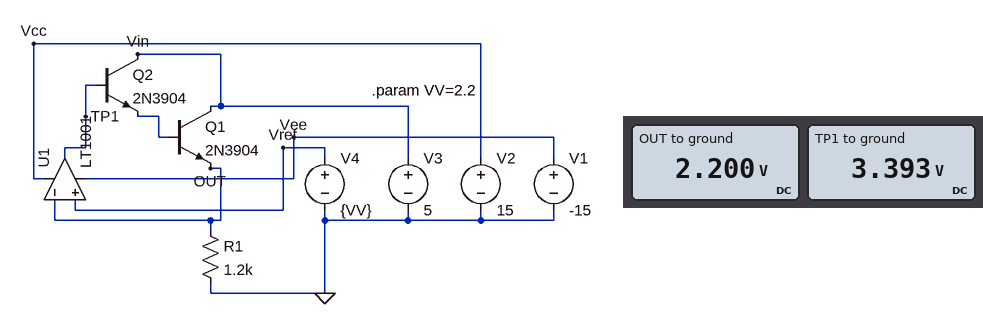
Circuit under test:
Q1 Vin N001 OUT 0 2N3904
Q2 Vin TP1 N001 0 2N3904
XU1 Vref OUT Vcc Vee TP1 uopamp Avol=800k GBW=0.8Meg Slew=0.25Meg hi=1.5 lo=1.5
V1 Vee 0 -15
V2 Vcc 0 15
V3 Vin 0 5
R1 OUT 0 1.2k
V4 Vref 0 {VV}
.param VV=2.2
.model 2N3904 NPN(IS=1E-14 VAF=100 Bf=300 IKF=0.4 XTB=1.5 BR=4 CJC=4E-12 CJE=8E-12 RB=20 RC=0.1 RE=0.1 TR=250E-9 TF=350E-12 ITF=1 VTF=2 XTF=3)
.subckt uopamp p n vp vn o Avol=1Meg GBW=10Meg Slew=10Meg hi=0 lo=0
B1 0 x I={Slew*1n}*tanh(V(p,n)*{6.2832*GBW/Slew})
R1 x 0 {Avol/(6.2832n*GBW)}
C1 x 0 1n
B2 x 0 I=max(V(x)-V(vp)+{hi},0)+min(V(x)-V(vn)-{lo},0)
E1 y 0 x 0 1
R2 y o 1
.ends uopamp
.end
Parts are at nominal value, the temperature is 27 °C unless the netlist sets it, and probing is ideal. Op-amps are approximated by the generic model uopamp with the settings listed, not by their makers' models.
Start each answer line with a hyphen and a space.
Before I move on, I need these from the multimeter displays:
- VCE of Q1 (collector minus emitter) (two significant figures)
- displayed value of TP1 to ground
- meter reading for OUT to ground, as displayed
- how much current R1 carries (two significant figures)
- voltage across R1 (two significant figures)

- 2.8 V
- 3.393 V
- 2.200 V
- 1.8 mA
- 2.2 V
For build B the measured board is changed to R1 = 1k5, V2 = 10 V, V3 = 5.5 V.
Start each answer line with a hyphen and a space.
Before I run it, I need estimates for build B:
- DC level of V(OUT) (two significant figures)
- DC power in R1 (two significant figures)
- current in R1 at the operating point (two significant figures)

- 2.2 V
- 3.2 mW
- 1.5 mA
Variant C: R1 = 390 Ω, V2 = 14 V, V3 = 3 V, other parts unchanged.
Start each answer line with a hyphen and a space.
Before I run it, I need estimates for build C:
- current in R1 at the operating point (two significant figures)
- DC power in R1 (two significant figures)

- 5.6 mA
- 12 mW
